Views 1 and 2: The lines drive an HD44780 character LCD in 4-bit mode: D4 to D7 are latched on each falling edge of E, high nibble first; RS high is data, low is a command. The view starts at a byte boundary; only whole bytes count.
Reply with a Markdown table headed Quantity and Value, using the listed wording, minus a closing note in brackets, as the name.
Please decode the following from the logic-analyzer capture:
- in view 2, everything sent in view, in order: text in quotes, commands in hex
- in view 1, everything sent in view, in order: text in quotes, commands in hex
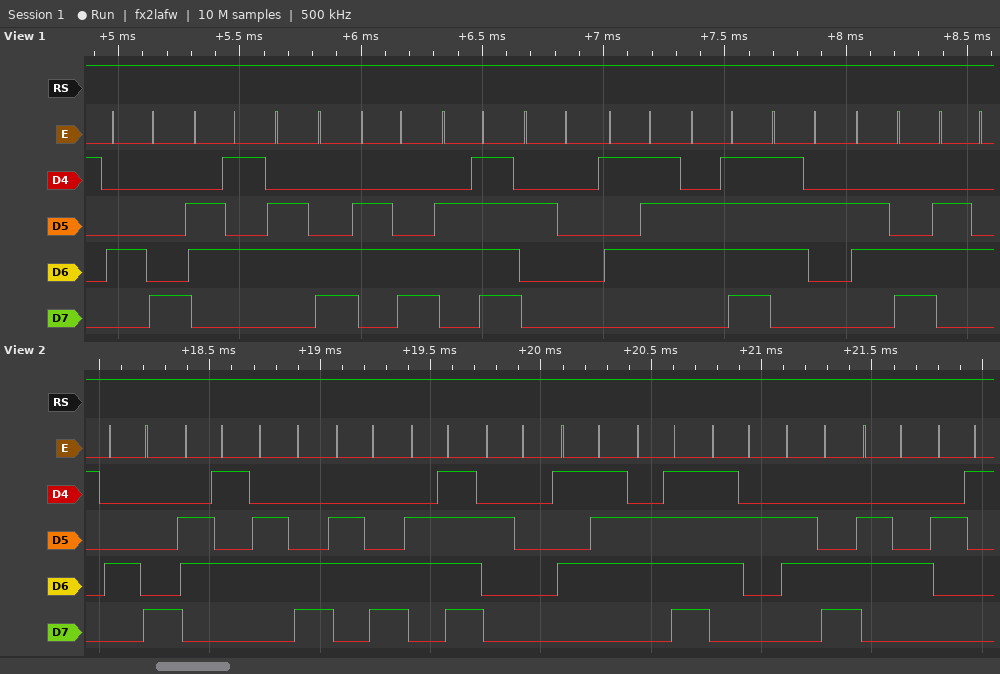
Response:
| Quantity | Value |
|---|---|
| in view 2, everything sent in view, in order: text in quotes, commands in hex | "Hello World!" |
| in view 1, everything sent in view, in order: text in quotes, commands in hex | "Hello World" |
